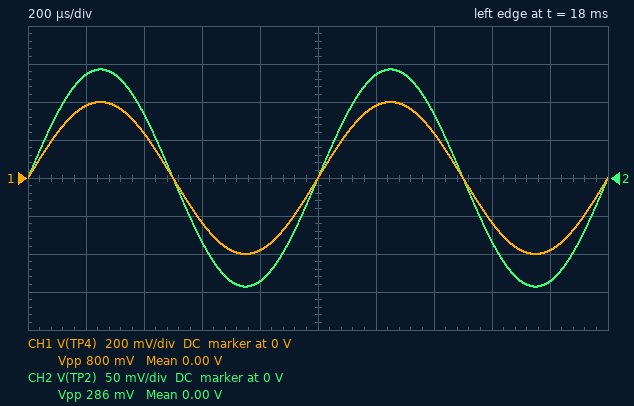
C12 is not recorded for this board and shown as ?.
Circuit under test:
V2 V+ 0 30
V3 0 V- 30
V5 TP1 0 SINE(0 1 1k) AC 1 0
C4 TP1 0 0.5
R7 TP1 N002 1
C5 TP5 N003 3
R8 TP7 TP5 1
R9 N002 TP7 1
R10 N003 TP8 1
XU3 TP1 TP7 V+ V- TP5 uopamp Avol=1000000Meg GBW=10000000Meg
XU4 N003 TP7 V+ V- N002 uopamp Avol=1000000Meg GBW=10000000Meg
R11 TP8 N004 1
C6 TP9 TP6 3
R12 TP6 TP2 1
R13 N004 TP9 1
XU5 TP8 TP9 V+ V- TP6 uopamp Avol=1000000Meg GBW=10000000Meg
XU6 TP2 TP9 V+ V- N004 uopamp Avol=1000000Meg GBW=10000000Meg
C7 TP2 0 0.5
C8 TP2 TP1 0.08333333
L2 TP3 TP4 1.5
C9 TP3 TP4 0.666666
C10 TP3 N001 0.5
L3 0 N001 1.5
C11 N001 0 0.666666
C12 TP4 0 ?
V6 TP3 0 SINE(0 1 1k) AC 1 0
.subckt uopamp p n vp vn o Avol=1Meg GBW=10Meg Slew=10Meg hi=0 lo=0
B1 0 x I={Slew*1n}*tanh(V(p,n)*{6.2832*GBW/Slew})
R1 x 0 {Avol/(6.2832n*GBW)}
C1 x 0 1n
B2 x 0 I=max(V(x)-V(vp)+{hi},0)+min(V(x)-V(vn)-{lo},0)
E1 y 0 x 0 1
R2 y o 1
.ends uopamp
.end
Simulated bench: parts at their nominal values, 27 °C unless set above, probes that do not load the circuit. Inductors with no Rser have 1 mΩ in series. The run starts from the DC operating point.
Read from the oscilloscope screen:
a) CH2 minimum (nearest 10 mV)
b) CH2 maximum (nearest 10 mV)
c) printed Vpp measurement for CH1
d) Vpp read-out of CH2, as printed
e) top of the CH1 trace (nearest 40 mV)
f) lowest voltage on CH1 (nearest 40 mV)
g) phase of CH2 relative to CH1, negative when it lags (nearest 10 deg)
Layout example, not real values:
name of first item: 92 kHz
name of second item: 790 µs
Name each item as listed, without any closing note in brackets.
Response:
CH2 minimum: -140 mV
CH2 maximum: 140 mV
printed Vpp measurement for CH1: 800 mV
Vpp read-out of CH2, as printed: 286 mV
top of the CH1 trace: 400 mV
lowest voltage on CH1: -400 mV
phase of CH2 relative to CH1, negative when it lags: 0 deg
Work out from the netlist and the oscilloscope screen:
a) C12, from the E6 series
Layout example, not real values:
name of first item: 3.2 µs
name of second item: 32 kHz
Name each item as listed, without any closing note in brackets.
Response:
C12, from the E6 series: 1 F
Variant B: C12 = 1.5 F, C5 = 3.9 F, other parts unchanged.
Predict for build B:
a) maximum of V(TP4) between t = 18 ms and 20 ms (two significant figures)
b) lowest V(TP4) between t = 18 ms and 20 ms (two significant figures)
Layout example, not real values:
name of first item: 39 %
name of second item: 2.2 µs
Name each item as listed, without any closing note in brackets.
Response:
maximum of V(TP4) between t = 18 ms and 20 ms: 310 mV
lowest V(TP4) between t = 18 ms and 20 ms: -310 mV
